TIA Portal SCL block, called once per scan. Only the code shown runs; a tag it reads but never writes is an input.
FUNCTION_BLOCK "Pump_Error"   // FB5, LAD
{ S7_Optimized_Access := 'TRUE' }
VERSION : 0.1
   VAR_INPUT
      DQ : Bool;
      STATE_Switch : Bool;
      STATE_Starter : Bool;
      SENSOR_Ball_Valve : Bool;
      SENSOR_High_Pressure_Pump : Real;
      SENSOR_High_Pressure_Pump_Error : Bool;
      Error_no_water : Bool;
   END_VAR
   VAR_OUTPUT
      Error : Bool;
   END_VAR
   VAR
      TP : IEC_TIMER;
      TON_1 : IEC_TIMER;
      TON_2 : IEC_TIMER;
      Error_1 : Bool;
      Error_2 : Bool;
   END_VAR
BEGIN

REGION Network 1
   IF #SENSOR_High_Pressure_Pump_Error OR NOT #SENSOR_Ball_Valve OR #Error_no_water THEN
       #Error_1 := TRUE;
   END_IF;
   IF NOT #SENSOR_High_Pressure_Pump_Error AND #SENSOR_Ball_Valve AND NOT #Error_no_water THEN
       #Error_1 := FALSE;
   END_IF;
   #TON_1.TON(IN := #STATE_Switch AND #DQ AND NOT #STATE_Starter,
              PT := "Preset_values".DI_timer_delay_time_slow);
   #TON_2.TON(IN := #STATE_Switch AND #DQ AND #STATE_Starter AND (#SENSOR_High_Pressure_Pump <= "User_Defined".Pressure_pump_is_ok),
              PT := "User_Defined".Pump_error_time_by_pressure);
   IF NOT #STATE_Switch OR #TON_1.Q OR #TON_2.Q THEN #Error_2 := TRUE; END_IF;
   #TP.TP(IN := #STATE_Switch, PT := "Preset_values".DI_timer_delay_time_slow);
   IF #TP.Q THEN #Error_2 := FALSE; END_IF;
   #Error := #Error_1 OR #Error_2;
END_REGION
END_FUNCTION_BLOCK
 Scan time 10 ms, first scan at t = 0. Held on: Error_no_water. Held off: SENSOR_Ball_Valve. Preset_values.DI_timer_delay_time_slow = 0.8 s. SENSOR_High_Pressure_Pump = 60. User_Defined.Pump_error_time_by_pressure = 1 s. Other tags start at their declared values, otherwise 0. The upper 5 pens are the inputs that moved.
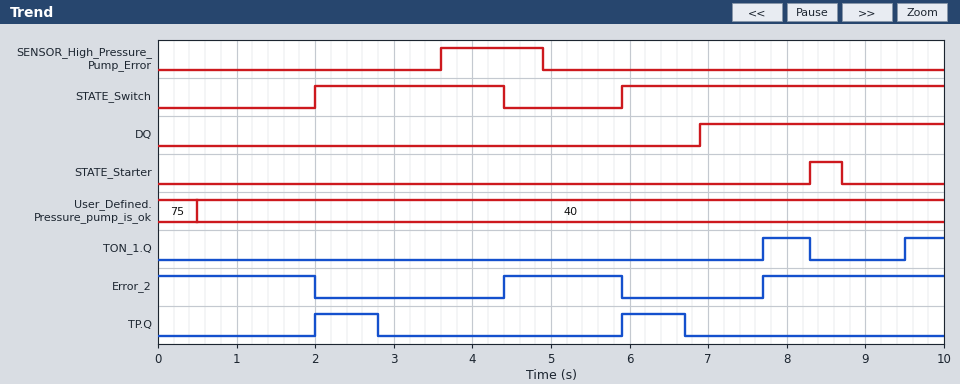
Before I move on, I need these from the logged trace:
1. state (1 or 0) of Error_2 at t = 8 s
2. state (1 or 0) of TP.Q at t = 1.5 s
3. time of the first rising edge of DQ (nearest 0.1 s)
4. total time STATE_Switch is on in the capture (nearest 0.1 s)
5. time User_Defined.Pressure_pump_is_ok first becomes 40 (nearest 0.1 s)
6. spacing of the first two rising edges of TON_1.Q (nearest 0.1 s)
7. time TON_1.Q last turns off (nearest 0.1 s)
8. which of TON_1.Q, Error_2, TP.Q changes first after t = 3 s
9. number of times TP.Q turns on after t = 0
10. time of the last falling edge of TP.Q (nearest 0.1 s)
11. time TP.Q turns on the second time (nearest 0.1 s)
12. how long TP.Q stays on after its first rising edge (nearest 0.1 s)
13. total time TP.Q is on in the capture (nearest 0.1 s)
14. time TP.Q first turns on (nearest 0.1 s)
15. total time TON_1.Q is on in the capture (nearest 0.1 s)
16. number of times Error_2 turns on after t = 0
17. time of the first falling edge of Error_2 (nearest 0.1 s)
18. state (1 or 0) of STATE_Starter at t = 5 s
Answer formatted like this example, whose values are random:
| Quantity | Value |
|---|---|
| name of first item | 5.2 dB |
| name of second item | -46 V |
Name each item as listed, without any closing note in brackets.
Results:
| Quantity | Value |
|---|---|
| state (1 or 0) of Error_2 at t = 8 s | 1 |
| state (1 or 0) of TP.Q at t = 1.5 s | 0 |
| time of the first rising edge of DQ | 6.9 s |
| total time STATE_Switch is on in the capture | 6.5 s |
| time User_Defined.Pressure_pump_is_ok first becomes 40 | 0.5 s |
| spacing of the first two rising edges of TON_1.Q | 1.8 s |
| time TON_1.Q last turns off | 8.3 s |
| which of TON_1.Q, Error_2, TP.Q changes first after t = 3 s | Error_2 |
| number of times TP.Q turns on after t = 0 | 2 |
| time of the last falling edge of TP.Q | 6.7 s |
| time TP.Q turns on the second time | 5.9 s |
| how long TP.Q stays on after its first rising edge | 0.8 s |
| total time TP.Q is on in the capture | 1.6 s |
| time TP.Q first turns on | 2.0 s |
| total time TON_1.Q is on in the capture | 1.1 s |
| number of times Error_2 turns on after t = 0 | 2 |
| time of the first falling edge of Error_2 | 2.0 s |
| state (1 or 0) of STATE_Starter at t = 5 s | 0 |
